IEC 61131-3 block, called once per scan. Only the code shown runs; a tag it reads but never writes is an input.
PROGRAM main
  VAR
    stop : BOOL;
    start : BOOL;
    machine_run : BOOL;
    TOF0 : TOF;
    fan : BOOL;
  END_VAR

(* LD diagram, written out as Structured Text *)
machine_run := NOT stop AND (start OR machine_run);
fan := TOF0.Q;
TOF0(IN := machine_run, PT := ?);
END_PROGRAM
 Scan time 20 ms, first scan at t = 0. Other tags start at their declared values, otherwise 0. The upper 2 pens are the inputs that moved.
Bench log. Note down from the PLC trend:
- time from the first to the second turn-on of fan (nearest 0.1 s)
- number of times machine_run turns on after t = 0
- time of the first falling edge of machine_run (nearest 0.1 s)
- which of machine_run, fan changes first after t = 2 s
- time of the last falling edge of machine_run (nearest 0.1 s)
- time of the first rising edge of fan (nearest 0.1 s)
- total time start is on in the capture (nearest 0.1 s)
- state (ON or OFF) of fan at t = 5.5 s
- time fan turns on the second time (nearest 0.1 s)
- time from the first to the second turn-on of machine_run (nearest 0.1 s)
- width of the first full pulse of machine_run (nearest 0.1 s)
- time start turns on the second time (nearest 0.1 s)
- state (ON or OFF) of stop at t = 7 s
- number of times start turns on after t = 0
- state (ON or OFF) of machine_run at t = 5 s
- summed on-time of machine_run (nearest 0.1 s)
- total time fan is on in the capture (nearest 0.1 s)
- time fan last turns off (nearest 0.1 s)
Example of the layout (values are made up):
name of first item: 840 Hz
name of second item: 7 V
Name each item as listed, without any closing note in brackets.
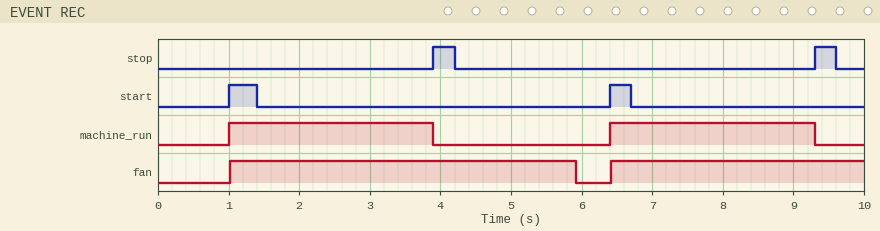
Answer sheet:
time from the first to the second turn-on of fan: 5.4 s
number of times machine_run turns on after t = 0: 2
time of the first falling edge of machine_run: 3.9 s
which of machine_run, fan changes first after t = 2 s: machine_run
time of the last falling edge of machine_run: 9.3 s
time of the first rising edge of fan: 1.0 s
total time start is on in the capture: 0.7 s
state (ON or OFF) of fan at t = 5.5 s: ON
time fan turns on the second time: 6.4 s
time from the first to the second turn-on of machine_run: 5.4 s
width of the first full pulse of machine_run: 2.9 s
time start turns on the second time: 6.4 s
state (ON or OFF) of stop at t = 7 s: OFF
number of times start turns on after t = 0: 2
state (ON or OFF) of machine_run at t = 5 s: OFF
summed on-time of machine_run: 5.8 s
total time fan is on in the capture: 8.5 s
time fan last turns off: 5.9 s
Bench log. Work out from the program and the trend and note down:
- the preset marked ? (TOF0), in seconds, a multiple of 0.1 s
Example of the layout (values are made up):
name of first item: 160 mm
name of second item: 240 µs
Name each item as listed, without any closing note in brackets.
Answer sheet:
the preset marked ? (TOF0), in seconds, a multiple of 0.1 s: 2.0 s
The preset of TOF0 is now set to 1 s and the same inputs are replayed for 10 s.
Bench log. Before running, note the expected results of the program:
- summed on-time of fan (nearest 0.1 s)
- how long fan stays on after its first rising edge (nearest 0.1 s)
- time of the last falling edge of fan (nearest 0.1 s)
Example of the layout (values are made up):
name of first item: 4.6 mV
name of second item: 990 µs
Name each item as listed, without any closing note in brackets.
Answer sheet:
summed on-time of fan: 7.5 s
how long fan stays on after its first rising edge: 3.9 s
time of the last falling edge of fan: 4.9 s
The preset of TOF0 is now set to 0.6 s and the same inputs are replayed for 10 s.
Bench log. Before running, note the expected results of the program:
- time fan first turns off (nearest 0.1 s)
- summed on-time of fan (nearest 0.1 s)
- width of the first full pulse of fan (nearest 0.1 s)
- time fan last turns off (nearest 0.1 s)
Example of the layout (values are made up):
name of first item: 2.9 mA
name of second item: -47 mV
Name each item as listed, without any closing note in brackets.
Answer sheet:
time fan first turns off: 4.5 s
summed on-time of fan: 7.0 s
width of the first full pulse of fan: 3.5 s
time fan last turns off: 9.9 s
